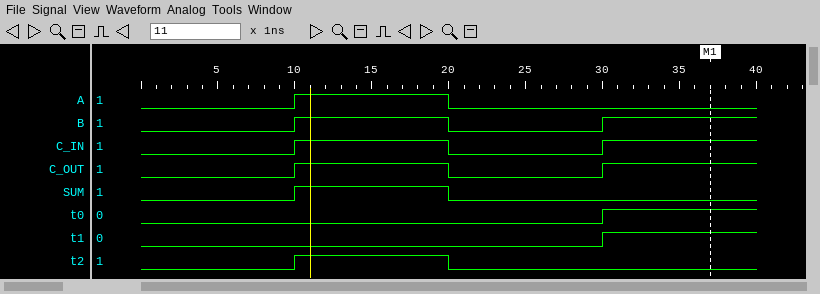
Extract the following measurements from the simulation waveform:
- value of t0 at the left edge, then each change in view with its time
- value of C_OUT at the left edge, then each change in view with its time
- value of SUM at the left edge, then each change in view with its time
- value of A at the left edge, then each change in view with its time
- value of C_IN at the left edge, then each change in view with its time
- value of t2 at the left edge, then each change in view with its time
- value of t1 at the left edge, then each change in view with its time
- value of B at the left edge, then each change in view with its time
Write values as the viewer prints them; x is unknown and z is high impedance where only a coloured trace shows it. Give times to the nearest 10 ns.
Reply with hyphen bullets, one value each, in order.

- 0, 1 at 30 ns
- 0, 1 at 10 ns, 0 at 20 ns, 1 at 30 ns
- 0, 1 at 10 ns, 0 at 20 ns
- 0, 1 at 10 ns, 0 at 20 ns
- 0, 1 at 10 ns, 0 at 20 ns, 1 at 30 ns
- 0, 1 at 10 ns, 0 at 20 ns
- 0, 1 at 30 ns
- 0, 1 at 10 ns, 0 at 20 ns, 1 at 30 ns
